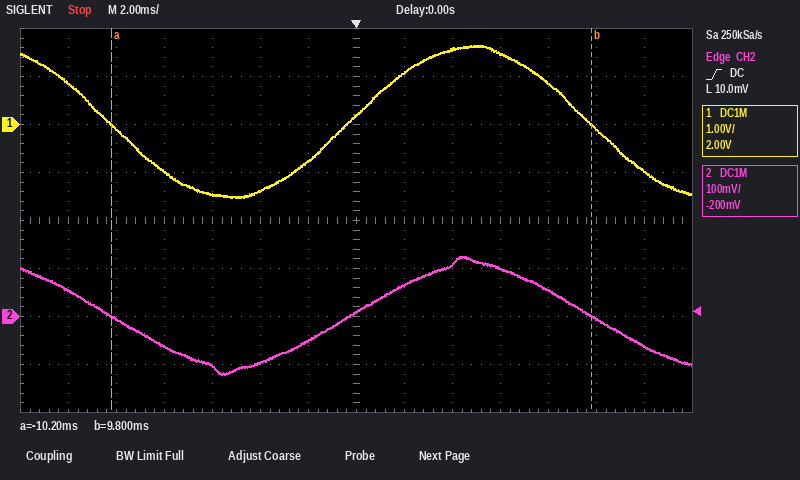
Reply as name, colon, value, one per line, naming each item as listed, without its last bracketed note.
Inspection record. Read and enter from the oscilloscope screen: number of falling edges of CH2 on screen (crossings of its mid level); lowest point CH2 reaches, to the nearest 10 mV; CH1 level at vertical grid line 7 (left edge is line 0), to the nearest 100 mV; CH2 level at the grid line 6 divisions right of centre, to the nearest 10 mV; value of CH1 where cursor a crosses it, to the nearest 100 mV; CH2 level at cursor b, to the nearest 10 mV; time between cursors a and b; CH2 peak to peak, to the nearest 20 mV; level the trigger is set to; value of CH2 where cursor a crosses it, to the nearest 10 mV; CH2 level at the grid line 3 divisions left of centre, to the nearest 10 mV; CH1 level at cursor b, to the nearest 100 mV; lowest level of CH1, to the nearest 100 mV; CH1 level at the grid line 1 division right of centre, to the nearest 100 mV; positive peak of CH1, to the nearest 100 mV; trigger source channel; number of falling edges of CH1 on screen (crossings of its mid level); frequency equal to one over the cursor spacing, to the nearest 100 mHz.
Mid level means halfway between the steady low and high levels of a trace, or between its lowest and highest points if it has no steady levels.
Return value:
number of falling edges of CH2 on screen: 2
lowest point CH2 reaches, to the nearest 10 mV: -120 mV
CH1 level at vertical grid line 7 (left edge is line 0), to the nearest 100 mV: 200 mV
CH2 level at the grid line 6 divisions right of centre, to the nearest 10 mV: -60 mV
value of CH1 where cursor a crosses it, to the nearest 100 mV: 0.0 V
CH2 level at cursor b, to the nearest 10 mV: 0 mV
time between cursors a and b: 20.0 ms
CH2 peak to peak, to the nearest 20 mV: 240 mV
level the trigger is set to: 10.0 mV
value of CH2 where cursor a crosses it, to the nearest 10 mV: 0 mV
CH2 level at the grid line 3 divisions left of centre, to the nearest 10 mV: -100 mV
CH1 level at cursor b, to the nearest 100 mV: 0.0 V
lowest level of CH1, to the nearest 100 mV: -1.5 V
CH1 level at the grid line 1 division right of centre, to the nearest 100 mV: 1.1 V
positive peak of CH1, to the nearest 100 mV: 1.6 V
trigger source channel: CH2
number of falling edges of CH1 on screen: 2
frequency equal to one over the cursor spacing, to the nearest 100 mHz: 50.0 Hz
